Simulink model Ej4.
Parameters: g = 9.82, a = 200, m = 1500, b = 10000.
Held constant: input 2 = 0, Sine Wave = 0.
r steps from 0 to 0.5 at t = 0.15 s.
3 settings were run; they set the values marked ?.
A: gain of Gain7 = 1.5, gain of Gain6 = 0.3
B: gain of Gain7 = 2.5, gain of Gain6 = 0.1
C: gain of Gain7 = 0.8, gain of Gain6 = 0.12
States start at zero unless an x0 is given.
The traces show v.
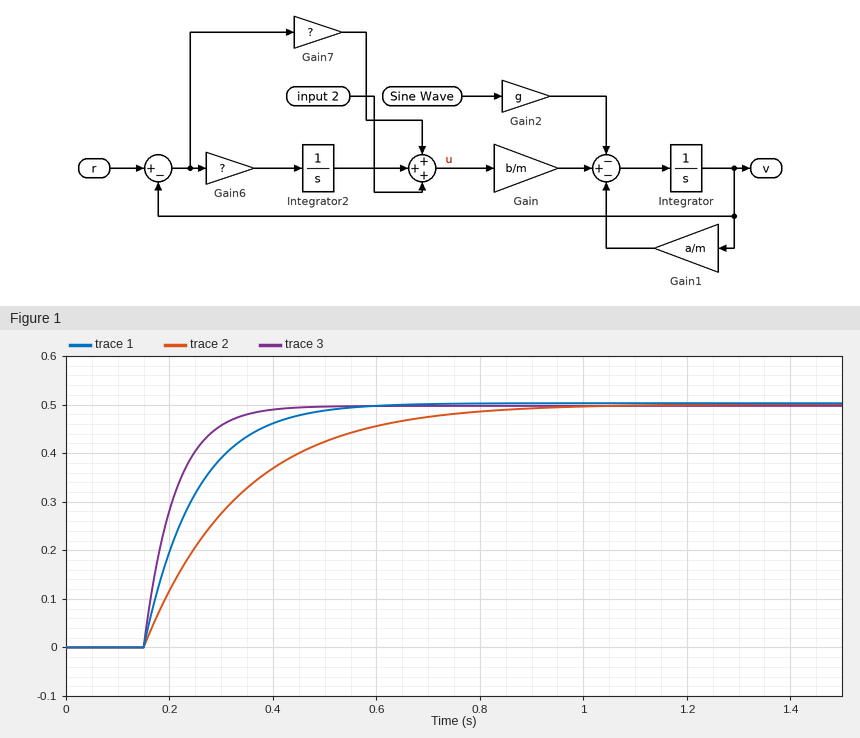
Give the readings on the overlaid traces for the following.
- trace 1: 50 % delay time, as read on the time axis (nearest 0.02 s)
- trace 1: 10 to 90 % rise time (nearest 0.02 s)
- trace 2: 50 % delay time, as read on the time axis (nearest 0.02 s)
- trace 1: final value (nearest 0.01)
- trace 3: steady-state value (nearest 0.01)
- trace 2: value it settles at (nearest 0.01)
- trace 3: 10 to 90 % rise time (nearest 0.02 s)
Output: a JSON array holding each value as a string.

["0.22 s", "0.22 s", "0.28 s", "0.50", "0.50", "0.50", "0.14 s"]
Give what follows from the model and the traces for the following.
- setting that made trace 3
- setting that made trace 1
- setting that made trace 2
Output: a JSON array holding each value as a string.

["B", "A", "C"]
